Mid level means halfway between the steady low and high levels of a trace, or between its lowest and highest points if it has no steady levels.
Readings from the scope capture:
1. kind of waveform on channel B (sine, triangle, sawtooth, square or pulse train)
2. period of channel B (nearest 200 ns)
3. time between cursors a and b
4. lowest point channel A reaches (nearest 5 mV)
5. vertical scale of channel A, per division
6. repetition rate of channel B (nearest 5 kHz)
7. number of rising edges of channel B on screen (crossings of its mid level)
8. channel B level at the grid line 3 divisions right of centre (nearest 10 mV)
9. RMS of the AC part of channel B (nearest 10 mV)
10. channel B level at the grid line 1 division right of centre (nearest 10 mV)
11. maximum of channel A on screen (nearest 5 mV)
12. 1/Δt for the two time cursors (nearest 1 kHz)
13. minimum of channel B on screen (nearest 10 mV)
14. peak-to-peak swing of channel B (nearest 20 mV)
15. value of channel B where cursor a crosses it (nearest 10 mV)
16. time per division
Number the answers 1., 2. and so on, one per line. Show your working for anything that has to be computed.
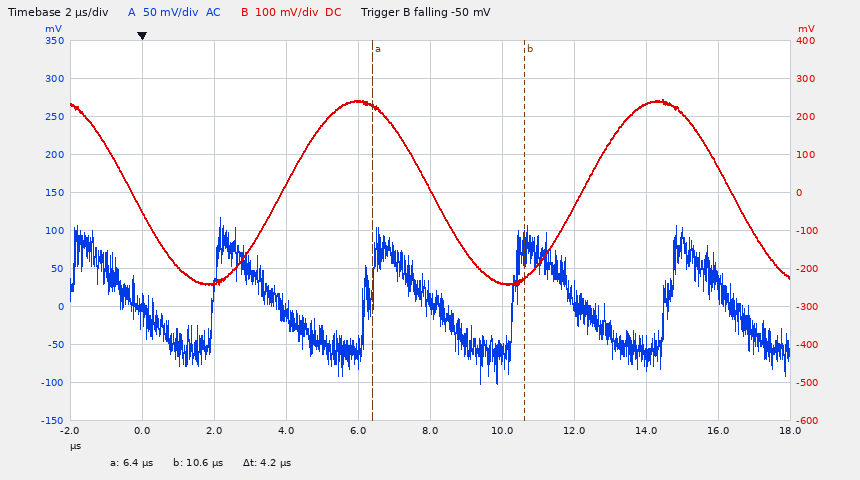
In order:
1. sine
2. 8.4 µs
3. 4.2 µs
4. -100 mV
5. 50 mV
6. 1 / 8.4 µs ≈ 119 kHz, so 120 kHz to the nearest 5 kHz
7. 2
8. 230 mV
9. 480 mV / (2√2) ≈ 170 mV
10. -240 mV
11. 115 mV
12. 1 / 4.2 µs ≈ 238 kHz
13. -240 mV
14. 480 mV
15. 230 mV
16. 2 µs
